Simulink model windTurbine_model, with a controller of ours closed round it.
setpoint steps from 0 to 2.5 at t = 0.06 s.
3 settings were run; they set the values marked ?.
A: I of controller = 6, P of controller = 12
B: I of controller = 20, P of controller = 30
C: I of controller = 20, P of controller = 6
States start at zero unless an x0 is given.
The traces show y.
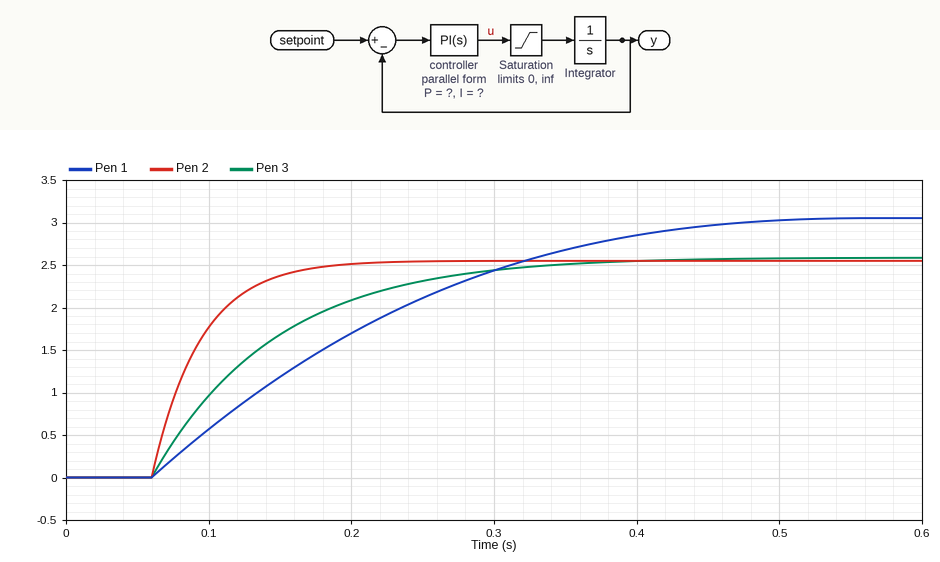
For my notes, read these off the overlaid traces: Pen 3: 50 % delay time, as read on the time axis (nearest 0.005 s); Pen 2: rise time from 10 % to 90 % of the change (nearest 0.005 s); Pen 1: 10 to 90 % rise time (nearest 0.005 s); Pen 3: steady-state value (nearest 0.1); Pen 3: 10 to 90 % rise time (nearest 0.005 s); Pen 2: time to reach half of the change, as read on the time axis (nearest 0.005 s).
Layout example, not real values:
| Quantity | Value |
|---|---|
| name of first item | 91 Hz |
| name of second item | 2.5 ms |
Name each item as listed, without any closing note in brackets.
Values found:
| Quantity | Value |
|---|---|
| Pen 3: 50 % delay time, as read on the time axis | 0.120 s |
| Pen 2: rise time from 10 % to 90 % of the change | 0.075 s |
| Pen 1: 10 to 90 % rise time | 0.285 s |
| Pen 3: steady-state value | 2.6 |
| Pen 3: 10 to 90 % rise time | 0.185 s |
| Pen 2: time to reach half of the change, as read on the time axis | 0.085 s |
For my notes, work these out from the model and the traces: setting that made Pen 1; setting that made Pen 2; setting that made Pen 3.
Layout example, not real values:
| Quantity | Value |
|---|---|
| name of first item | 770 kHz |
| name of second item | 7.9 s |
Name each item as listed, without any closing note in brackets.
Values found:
| Quantity | Value |
|---|---|
| setting that made Pen 1 | C |
| setting that made Pen 2 | B |
| setting that made Pen 3 | A |
